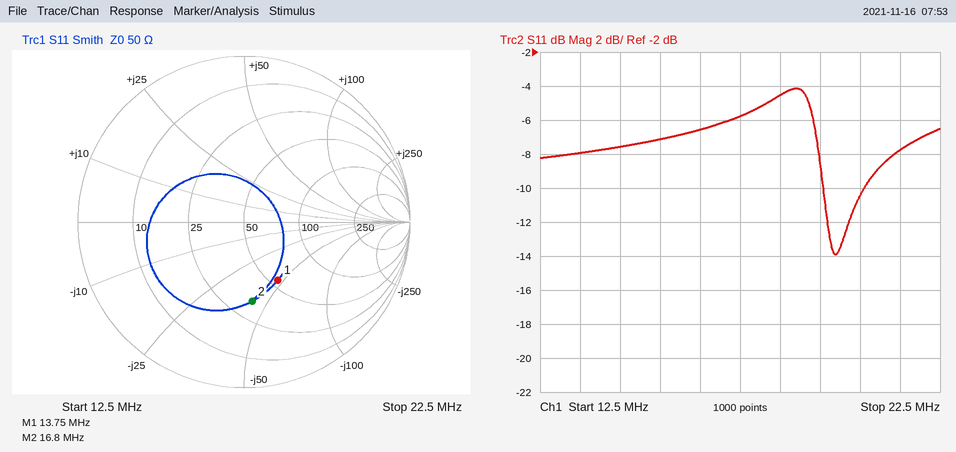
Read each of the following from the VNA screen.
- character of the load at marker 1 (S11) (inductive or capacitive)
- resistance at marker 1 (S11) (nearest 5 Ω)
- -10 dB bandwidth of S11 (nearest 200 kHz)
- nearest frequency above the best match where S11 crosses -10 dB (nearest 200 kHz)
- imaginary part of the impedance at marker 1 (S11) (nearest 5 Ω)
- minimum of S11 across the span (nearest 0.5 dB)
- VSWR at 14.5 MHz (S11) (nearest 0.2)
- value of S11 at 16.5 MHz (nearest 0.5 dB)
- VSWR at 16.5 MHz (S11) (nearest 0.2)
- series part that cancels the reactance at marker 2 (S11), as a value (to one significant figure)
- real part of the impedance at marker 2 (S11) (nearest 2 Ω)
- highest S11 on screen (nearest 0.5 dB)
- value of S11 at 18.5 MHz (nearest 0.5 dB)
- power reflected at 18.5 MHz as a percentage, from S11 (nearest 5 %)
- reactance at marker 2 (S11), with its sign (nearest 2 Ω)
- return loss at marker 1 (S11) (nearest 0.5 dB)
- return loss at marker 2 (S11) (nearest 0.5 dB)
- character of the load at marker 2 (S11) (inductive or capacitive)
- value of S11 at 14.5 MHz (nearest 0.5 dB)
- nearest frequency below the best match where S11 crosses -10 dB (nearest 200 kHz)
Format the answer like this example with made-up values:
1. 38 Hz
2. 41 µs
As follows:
1. capacitive
2. 55 Ω
3. 1.0 MHz
4. 20.6 MHz
5. -45 Ω
6. -14.0 dB
7. 2.4
8. -6.5 dB
9. 2.8
10. 400 nH
11. 34 Ω
12. -4.0 dB
13. -4.5 dB
14. 35 %
15. -42 Ω
16. 8.0 dB
17. 6.5 dB
18. capacitive
19. -7.5 dB
20. 19.6 MHz
